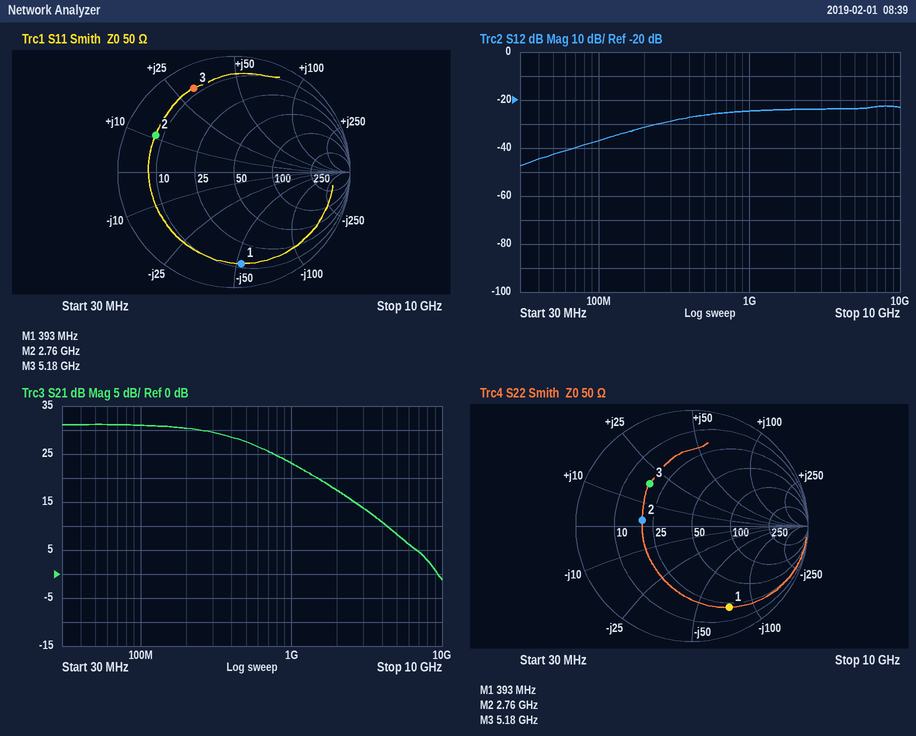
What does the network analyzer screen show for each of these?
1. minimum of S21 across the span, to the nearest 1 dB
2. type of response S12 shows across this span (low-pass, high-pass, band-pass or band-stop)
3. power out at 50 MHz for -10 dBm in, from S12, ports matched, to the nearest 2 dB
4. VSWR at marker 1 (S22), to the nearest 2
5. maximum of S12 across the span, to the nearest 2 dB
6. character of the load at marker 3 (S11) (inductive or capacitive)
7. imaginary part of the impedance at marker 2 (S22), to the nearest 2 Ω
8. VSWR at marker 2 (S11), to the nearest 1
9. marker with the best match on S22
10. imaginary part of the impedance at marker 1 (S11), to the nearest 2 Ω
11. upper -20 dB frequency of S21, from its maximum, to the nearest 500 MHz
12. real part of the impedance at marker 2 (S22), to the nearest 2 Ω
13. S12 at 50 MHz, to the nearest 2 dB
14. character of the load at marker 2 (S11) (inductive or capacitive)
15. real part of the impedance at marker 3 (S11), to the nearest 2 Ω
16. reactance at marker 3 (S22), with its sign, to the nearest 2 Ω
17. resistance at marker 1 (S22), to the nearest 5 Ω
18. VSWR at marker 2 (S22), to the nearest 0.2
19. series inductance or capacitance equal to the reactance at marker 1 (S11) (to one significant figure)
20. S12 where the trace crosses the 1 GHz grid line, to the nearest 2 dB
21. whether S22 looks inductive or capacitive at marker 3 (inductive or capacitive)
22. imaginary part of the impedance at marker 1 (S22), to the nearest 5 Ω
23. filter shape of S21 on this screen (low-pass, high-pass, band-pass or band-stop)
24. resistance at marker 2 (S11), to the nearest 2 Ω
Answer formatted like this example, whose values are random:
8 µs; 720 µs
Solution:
-1 dB; high-pass; -52 dBm; 8; -22 dB; inductive; +2 Ω; 7; marker 2; -52 Ω; 4.0 GHz; 20 Ω; -42 dB; inductive; 8 Ω; +18 Ω; 20 Ω; 2.6; 8 pF; -24 dB; inductive; -75 Ω; low-pass; 8 Ω
